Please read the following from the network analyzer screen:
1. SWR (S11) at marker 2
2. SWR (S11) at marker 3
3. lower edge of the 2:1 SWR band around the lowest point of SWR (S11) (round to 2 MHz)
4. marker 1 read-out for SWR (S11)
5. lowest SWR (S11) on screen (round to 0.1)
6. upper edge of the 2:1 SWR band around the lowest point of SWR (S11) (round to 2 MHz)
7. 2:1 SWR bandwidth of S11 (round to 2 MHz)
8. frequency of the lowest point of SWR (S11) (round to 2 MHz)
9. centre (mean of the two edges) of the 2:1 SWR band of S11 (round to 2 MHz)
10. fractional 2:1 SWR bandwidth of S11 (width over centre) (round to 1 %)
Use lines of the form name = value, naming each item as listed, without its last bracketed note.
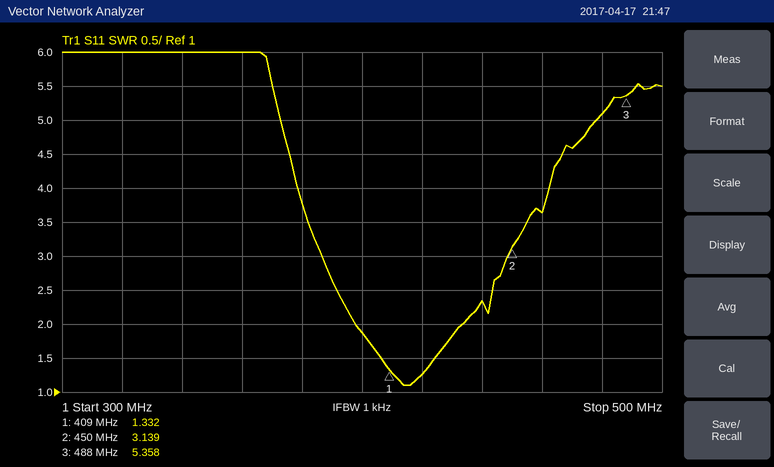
SWR (S11) at marker 2 = 3.139
SWR (S11) at marker 3 = 5.358
lower edge of the 2:1 SWR band around the lowest point of SWR (S11) = 398 MHz
marker 1 read-out for SWR = 1.332
lowest SWR (S11) on screen = 1.1
upper edge of the 2:1 SWR band around the lowest point of SWR (S11) = 434 MHz
2:1 SWR bandwidth of S11 = 36 MHz
frequency of the lowest point of SWR (S11) = 414 MHz
centre (mean of the two edges) of the 2:1 SWR band of S11 = 416 MHz
fractional 2:1 SWR bandwidth of S11 (width over centre) = 9 %
